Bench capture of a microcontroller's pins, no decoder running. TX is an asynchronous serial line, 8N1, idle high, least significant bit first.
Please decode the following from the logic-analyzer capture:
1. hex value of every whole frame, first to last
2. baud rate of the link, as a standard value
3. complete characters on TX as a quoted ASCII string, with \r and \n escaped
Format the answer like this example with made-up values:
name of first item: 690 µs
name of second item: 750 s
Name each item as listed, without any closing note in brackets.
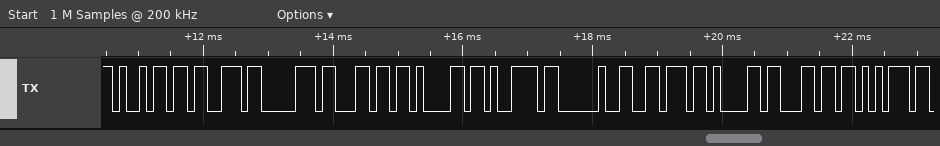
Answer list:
hex value of every whole frame, first to last: 0x69 0x73 0x70 0x6C 0x61 0x79 0x20 0x76 0x61 0x6C 0x75
baud rate of the link, as a standard value: 9600 baud
complete characters on TX as a quoted ASCII string, with \r and \n escaped: "isplay valu"
